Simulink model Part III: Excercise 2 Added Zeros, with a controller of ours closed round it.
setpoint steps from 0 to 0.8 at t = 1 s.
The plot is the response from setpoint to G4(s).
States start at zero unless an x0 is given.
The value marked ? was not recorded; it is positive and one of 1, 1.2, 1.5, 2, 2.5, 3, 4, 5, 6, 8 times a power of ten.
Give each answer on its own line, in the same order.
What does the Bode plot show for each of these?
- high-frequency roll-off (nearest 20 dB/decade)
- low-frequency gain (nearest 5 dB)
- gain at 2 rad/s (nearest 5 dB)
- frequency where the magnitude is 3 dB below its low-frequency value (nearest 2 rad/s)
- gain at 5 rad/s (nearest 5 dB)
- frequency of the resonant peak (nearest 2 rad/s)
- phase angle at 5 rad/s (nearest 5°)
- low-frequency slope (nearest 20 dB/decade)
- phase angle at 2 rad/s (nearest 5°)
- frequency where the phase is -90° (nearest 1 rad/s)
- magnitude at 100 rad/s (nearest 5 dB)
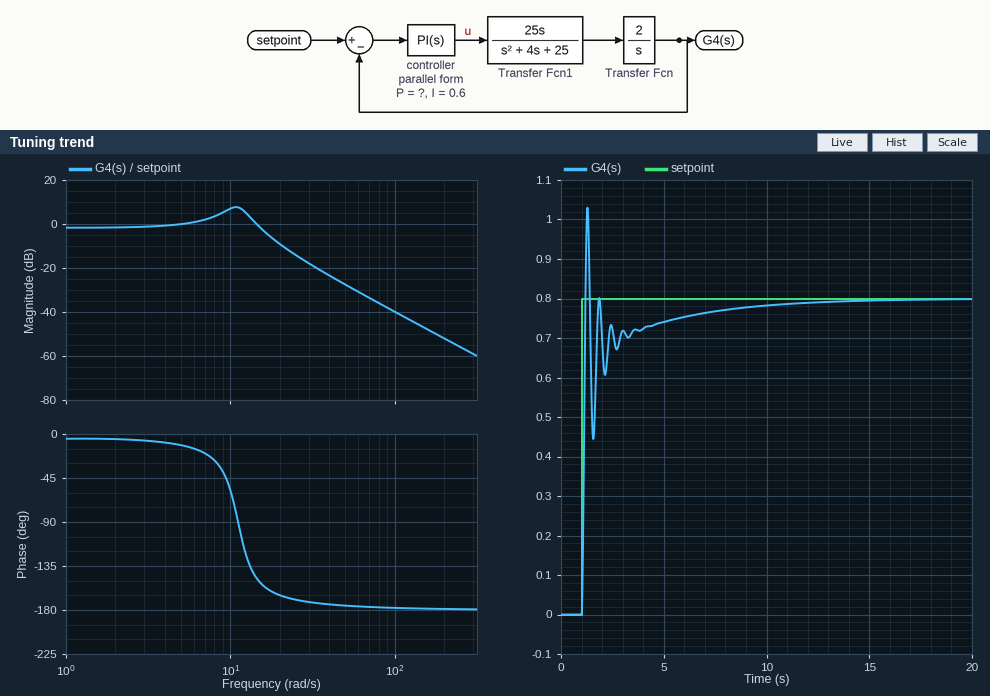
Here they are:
-40 dB/decade
0 dB
0 dB
16 rad/s
0 dB
10 rad/s
-10°
0 dB/decade
-5°
11 rad/s
-40 dB
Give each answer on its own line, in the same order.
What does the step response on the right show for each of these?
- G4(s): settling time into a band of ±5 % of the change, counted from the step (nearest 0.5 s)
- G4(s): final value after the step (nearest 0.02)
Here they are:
5.5 s
0.80
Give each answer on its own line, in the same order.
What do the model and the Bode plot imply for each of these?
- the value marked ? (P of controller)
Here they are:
2
